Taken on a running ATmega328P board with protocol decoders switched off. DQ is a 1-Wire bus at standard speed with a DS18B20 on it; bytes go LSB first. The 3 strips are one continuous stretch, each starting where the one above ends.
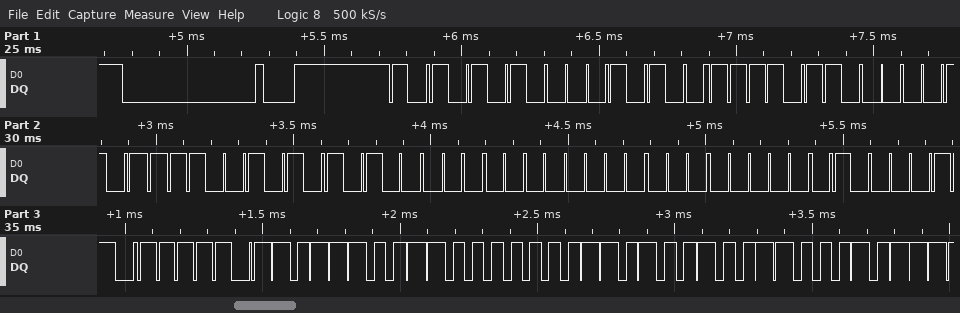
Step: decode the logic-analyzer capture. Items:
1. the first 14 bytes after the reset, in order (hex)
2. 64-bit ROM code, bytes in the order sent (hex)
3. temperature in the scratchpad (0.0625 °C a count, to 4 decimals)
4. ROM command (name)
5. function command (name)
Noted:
55 28 6F D0 53 05 00 00 C2 BE 9D 01 4B 46
28 6F D0 53 05 00 00 C2
25.8125 °C
Match ROM
Read Scratchpad
